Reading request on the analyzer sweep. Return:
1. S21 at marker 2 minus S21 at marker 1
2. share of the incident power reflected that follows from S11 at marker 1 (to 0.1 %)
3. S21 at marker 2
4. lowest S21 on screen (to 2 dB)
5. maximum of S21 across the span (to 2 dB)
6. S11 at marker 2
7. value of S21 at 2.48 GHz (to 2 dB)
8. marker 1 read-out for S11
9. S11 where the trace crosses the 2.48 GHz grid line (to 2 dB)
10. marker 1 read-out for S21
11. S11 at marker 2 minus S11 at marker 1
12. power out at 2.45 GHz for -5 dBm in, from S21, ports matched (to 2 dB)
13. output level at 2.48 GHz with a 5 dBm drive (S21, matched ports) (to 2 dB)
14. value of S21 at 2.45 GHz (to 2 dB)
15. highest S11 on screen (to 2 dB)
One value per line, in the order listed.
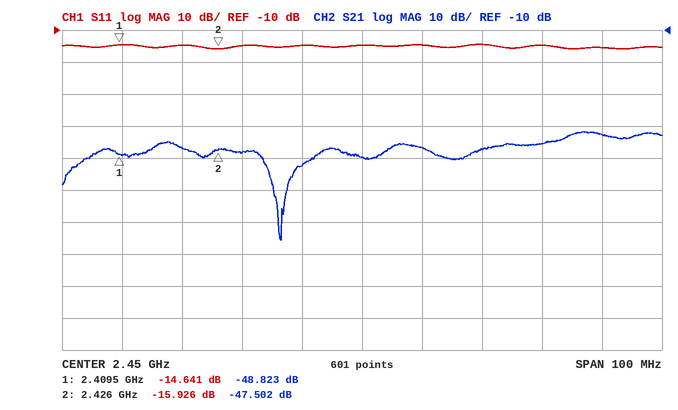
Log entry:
1.321 dB
3.4 %
-47.502 dB
-76 dB
-42 dB
-15.926 dB
-46 dB
-14.641 dB
-14 dB
-48.823 dB
-1.285 dB
-54 dBm
-40 dBm
-50 dB
-14 dB
